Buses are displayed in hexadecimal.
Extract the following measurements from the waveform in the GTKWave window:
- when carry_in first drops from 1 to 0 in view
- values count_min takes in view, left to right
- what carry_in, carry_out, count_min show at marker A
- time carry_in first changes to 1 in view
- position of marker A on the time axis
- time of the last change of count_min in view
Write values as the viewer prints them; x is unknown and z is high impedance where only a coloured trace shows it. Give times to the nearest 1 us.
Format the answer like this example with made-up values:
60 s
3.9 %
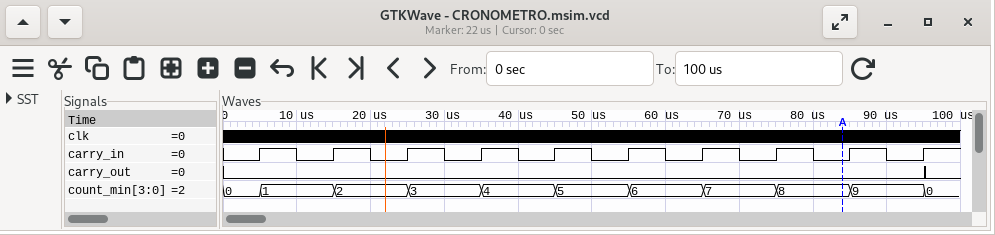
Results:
10 us
0, 1, 2, 3, 4, 5, 6, 7, 8, 9, 0
carry_in=0, carry_out=0, count_min=8
5 us
84 us
95 us
